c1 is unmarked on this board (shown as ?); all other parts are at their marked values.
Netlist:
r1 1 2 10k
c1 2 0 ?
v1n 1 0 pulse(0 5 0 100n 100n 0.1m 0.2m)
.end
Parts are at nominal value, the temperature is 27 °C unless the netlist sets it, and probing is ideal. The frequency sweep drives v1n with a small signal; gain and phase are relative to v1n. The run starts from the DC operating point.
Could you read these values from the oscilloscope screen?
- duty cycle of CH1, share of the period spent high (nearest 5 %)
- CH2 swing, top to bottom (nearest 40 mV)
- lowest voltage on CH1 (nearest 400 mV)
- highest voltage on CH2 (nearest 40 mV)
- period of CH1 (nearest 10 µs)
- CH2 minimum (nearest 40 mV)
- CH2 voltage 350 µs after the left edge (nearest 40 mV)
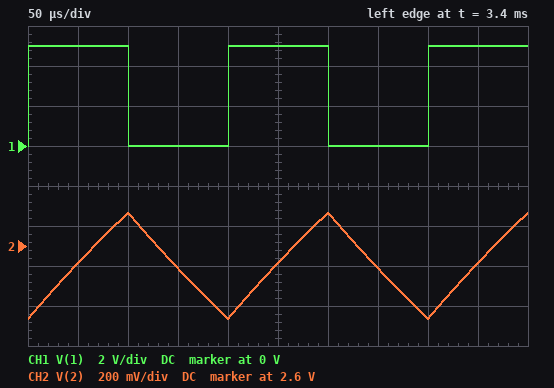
50 %
520 mV
0 V
2.76 V
200 µs
2.24 V
2.48 V
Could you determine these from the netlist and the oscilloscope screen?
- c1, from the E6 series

47 nF
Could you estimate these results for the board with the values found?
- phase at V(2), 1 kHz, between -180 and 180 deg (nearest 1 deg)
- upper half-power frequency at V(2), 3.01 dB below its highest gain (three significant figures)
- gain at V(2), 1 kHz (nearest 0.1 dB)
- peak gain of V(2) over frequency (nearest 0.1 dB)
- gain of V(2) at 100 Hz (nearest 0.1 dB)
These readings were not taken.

-71 deg
339 Hz
-9.9 dB
0 dB
-0.4 dB
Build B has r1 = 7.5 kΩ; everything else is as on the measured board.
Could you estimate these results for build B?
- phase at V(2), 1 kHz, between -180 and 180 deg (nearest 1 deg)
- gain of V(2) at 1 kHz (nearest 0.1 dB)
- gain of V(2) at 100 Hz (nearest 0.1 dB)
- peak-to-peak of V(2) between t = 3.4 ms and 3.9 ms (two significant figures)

-66 deg
-7.7 dB
-0.2 dB
700 mV
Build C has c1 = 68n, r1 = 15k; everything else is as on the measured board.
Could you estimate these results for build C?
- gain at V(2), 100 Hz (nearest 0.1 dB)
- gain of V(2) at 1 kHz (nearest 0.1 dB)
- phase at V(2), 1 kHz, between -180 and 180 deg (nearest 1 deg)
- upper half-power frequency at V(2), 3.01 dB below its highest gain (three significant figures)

-1.5 dB
-16.2 dB
-81 deg
156 Hz
